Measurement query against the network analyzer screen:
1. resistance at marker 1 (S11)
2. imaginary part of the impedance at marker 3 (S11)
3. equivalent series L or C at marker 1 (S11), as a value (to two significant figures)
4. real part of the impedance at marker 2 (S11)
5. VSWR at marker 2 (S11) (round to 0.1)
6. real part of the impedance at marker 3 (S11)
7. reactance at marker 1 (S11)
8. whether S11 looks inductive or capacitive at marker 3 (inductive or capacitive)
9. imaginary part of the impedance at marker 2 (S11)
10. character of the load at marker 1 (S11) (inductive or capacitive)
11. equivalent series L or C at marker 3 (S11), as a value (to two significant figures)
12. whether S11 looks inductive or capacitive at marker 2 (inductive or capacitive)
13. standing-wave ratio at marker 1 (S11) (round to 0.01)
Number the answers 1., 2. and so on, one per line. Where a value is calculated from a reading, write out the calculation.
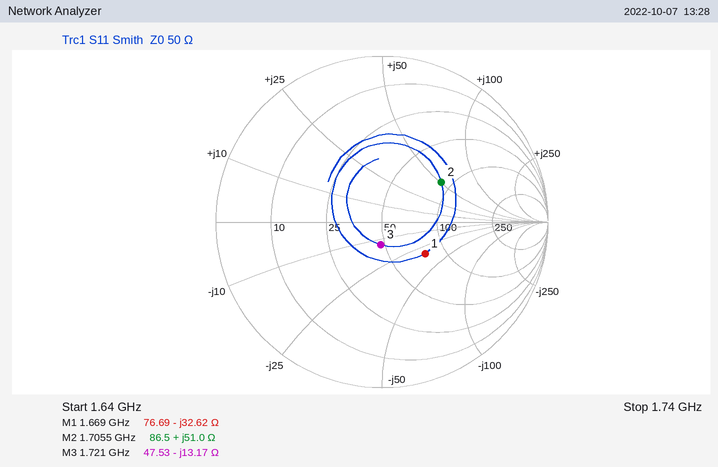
1. 76.69 Ω
2. -13.17 Ω
3. C = 1/(2π × 1.669 GHz × 32.62 Ω) ≈ 2.9 pF
4. 86.5 Ω
5. 2.5
6. 47.53 Ω
7. -32.62 Ω
8. capacitive
9. +51.0 Ω
10. capacitive
11. C = 1/(2π × 1.721 GHz × 13.17 Ω) ≈ 7.0 pF
12. inductive
13. 1.95
